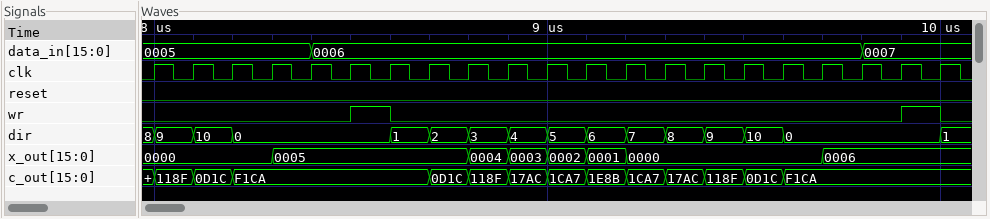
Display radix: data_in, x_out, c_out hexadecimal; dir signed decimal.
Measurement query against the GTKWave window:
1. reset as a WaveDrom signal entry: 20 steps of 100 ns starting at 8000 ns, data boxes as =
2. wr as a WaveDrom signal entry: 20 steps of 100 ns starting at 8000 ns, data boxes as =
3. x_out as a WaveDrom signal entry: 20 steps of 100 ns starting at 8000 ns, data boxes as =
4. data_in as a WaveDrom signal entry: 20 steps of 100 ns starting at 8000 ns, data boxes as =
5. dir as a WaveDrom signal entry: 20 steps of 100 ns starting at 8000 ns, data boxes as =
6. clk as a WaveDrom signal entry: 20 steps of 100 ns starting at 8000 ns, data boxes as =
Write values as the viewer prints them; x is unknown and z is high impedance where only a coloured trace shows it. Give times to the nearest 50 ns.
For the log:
{name: 'reset', wave: '0...................'}
{name: 'wr', wave: '0....10............1'}
{name: 'x_out', wave: '=..=....=====....=..', data: '0000 0005 0004 0003 0002 0001 0000 0006'}
{name: 'data_in', wave: '=...=.............=.', data: '0005 0006 0007'}
{name: 'dir', wave: '===...===========...', data: '9 10 0 1 2 3 4 5 6 7 8 9 10 0'}
{name: 'clk', wave: 'p...................'}
